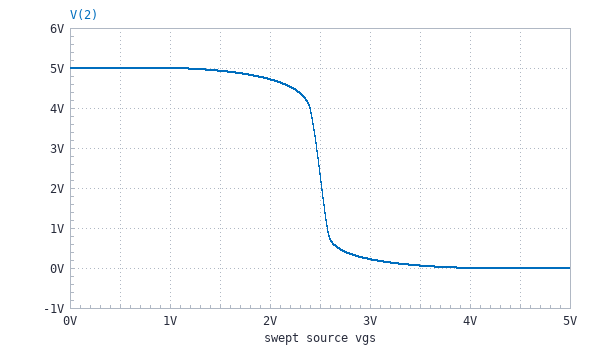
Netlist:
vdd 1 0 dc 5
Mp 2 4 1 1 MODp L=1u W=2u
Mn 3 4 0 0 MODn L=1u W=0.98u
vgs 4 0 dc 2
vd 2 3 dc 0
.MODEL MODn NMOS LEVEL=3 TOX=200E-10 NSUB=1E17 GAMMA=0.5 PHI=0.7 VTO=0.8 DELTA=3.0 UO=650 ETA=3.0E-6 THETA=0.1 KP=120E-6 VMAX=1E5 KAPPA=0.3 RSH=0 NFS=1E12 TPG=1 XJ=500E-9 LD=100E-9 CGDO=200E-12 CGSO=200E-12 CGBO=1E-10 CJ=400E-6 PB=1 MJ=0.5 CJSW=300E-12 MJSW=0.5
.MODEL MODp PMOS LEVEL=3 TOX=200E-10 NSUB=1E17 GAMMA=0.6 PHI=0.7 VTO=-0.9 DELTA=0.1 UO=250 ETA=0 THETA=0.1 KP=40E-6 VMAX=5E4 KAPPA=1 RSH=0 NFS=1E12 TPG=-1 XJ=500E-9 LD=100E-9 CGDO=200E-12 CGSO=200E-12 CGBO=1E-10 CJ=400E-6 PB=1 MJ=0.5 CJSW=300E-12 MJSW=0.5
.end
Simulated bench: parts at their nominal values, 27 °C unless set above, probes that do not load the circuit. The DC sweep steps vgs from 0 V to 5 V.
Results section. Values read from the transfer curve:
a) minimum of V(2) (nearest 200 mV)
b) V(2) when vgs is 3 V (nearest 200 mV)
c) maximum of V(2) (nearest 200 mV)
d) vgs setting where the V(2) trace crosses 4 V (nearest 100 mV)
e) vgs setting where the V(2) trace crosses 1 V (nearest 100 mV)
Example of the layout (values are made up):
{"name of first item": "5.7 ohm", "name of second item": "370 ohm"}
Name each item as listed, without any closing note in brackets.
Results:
{"minimum of V(2)": "0 V", "V(2) when vgs is 3 V": "200 mV", "maximum of V(2)": "5.0 V", "vgs setting where the V(2) trace crosses 4 V": "2.4 V", "vgs setting where the V(2) trace crosses 1 V": "2.6 V"}
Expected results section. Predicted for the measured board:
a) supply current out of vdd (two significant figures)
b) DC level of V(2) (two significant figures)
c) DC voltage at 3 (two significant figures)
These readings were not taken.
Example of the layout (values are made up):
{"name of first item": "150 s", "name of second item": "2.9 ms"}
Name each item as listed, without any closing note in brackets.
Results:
{"supply current out of vdd": "40 µA", "DC level of V(2)": "4.7 V", "DC voltage at 3": "4.7 V"}
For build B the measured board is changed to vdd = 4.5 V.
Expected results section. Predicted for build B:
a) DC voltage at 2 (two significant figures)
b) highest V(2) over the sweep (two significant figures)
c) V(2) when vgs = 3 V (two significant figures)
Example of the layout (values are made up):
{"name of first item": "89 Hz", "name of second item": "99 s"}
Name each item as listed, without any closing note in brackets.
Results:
{"DC voltage at 2": "4.1 V", "highest V(2) over the sweep": "4.5 V", "V(2) when vgs = 3 V": "74 mV"}
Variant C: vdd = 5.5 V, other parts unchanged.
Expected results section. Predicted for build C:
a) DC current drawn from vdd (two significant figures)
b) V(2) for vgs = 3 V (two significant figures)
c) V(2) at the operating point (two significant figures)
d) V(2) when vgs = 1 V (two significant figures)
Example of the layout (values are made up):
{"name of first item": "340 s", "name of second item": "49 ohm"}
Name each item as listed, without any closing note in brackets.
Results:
{"DC current drawn from vdd": "41 µA", "V(2) for vgs = 3 V": "510 mV", "V(2) at the operating point": "5.3 V", "V(2) when vgs = 1 V": "5.5 V"}
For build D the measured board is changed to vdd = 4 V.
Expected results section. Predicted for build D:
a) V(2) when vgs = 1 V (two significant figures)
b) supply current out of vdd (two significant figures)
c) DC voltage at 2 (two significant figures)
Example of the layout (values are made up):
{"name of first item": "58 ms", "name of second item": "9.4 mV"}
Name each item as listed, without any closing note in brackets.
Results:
{"V(2) when vgs = 1 V": "4.0 V", "supply current out of vdd": "38 µA", "DC voltage at 2": "2.3 V"}
